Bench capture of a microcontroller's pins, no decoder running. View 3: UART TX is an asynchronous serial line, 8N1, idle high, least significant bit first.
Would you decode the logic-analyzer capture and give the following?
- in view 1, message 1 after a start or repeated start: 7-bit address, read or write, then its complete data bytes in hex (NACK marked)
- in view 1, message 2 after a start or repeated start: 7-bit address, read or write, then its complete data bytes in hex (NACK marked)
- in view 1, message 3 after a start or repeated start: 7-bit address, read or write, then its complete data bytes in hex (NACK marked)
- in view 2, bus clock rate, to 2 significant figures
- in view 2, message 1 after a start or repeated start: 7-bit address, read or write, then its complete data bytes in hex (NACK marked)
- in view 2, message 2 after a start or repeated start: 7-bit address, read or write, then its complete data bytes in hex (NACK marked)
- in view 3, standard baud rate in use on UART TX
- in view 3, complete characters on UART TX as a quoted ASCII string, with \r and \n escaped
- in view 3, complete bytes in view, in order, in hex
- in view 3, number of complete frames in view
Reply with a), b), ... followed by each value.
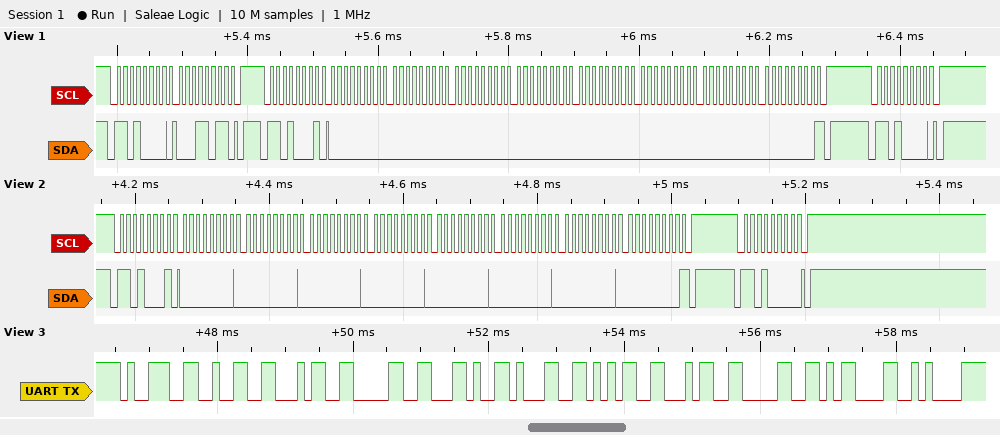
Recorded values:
a) 0x68 write: 1B
b) 0x68 read: 00 00 00 00 00 00 00 00 NACK
c) 0x68 write
d) 100 kHz
e) 0x68 read: 00 00 00 00 00 00 00 00 NACK
f) 0x68 write
g) 9600 baud
h) "9240,1540\r\n"
i) 0x39 0x32 0x34 0x30 0x2C 0x31 0x35 0x34 0x30 0x0D 0x0A
j) 11
